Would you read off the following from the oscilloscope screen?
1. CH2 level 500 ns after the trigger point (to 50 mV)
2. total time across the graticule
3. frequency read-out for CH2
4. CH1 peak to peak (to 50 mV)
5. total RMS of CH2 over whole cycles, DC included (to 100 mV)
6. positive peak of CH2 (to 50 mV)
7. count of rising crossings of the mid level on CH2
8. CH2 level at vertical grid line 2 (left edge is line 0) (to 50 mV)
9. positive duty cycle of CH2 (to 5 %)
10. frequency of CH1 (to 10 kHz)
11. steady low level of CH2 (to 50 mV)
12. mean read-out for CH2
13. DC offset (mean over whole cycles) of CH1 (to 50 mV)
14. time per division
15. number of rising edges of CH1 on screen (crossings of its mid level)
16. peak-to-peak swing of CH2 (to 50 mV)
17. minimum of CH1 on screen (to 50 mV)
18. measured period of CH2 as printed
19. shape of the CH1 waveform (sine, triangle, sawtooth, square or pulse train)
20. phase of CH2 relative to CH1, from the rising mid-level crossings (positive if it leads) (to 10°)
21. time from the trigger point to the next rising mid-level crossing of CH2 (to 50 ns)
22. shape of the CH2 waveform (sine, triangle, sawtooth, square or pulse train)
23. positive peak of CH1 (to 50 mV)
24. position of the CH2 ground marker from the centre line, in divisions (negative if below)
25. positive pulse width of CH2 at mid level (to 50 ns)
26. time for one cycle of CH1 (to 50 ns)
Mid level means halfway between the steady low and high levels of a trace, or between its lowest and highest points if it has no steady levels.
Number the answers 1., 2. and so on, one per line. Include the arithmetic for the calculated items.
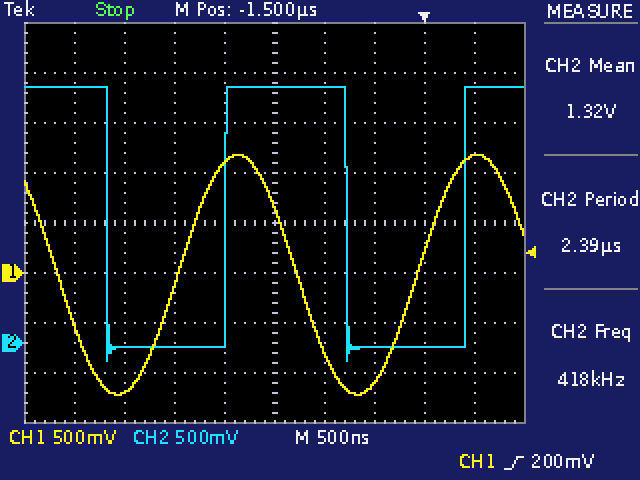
1. 2.55 V
2. 5 µs
3. 418 kHz
4. 1.20 V − (-1.20 V) = 2.40 V
5. √(0.5 × (2.55 V)² + 0.5 × (-50 mV)²) ≈ 1.8 V
6. 2.55 V
7. 2
8. -50 mV
9. 50 %
10. 1 / 2.40 µs ≈ 417 kHz, so 420 kHz to the nearest 10 kHz
11. -50 mV
12. 1.32 V
13. (1.20 V + (-1.20 V)) / 2 ≈ 0 mV
14. 500 ns
15. 2
16. 2.55 V − (-200 mV) = 2.75 V
17. -1.20 V
18. 2.39 µs
19. sine
20. -70°
21. 400 ns
22. square
23. 1.20 V
24. -2.4 div
25. 1.20 µs
26. 2.40 µs
